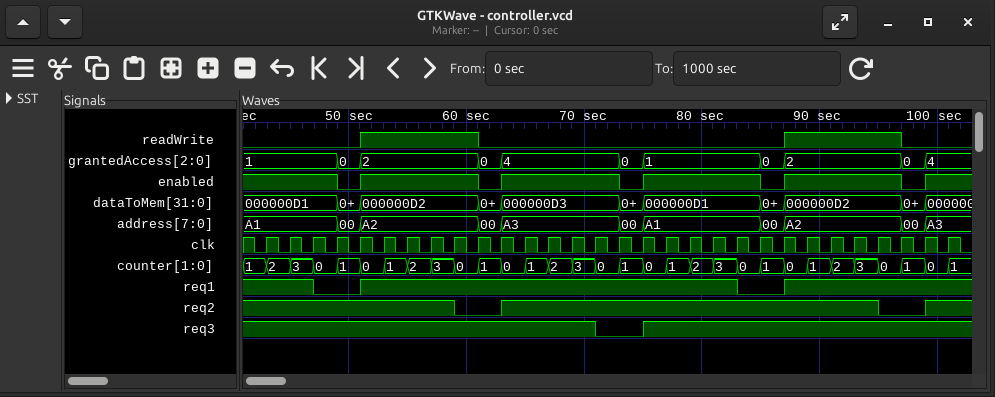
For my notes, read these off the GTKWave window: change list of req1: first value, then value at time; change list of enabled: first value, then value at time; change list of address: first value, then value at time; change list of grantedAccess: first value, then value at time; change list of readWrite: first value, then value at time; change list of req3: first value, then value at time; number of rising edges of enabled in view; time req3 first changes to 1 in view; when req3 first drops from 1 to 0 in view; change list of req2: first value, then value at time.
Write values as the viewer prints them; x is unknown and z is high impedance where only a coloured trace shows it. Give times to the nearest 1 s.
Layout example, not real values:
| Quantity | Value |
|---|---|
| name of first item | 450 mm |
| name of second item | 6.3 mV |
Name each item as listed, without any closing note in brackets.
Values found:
| Quantity | Value |
|---|---|
| change list of req1: first value, then value at time | 1, 0 at 47 s, 1 at 51 s, 0 at 83 s, 1 at 87 s |
| change list of enabled: first value, then value at time | 1, 0 at 49 s, 1 at 51 s, 0 at 61 s, 1 at 63 s, 0 at 73 s, 1 at 75 s, 0 at 85 s, 1 at 87 s, 0 at 97 s, 1 at 99 s |
| change list of address: first value, then value at time | A1, 00 at 49 s, A2 at 51 s, 00 at 61 s, A3 at 63 s, 00 at 73 s, A1 at 75 s, 00 at 85 s, A2 at 87 s, 00 at 97 s, A3 at 99 s |
| change list of grantedAccess: first value, then value at time | 1, 0 at 49 s, 2 at 51 s, 0 at 61 s, 4 at 63 s, 0 at 73 s, 1 at 75 s, 0 at 85 s, 2 at 87 s, 0 at 97 s, 4 at 99 s |
| change list of readWrite: first value, then value at time | 0, 1 at 51 s, 0 at 61 s, 1 at 87 s, 0 at 97 s |
| change list of req3: first value, then value at time | 1, 0 at 71 s, 1 at 75 s |
| number of rising edges of enabled in view | 5 |
| time req3 first changes to 1 in view | 75 s |
| when req3 first drops from 1 to 0 in view | 71 s |
| change list of req2: first value, then value at time | 1, 0 at 59 s, 1 at 63 s, 0 at 95 s, 1 at 99 s |
